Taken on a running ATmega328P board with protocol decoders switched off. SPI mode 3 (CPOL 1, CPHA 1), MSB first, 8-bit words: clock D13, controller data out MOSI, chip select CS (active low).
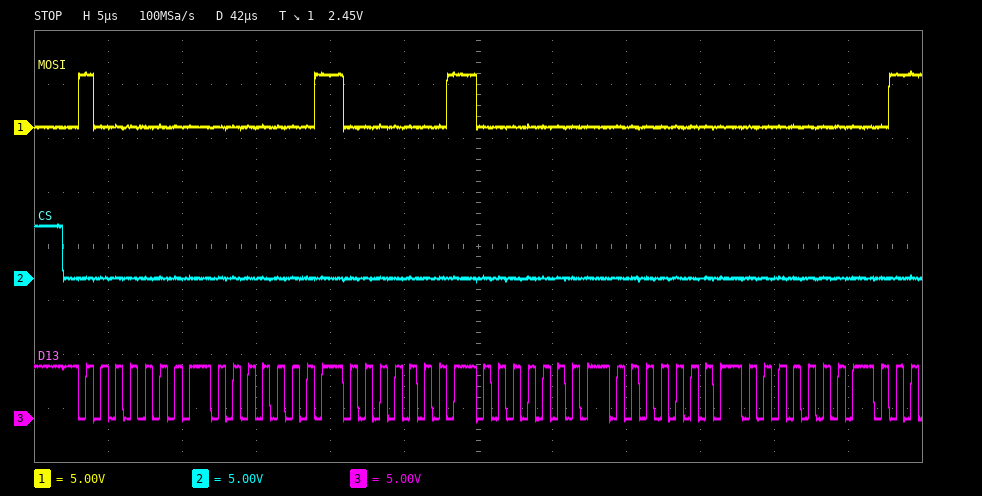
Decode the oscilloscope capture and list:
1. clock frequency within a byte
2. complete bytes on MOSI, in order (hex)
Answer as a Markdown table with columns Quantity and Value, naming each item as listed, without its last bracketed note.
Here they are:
| Quantity | Value |
|---|---|
| clock frequency within a byte | 1 MHz |
| complete bytes on MOSI, in order | 80 01 01 00 00 00 |
